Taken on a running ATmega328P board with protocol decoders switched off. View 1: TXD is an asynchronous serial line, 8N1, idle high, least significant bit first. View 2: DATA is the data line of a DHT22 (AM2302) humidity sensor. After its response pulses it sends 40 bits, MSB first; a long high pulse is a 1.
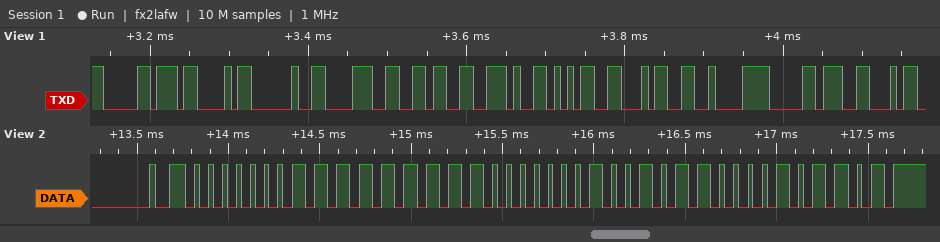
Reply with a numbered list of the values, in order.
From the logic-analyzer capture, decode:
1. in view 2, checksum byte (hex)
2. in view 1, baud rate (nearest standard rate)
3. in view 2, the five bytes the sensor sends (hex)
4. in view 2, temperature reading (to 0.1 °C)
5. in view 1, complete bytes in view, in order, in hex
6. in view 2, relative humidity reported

1. 0x2D
2. 115200 baud
3. 01 FF 01 2C 2D
4. 30.0 °C
5. B0 43 20 38 36 2E 35 34 C2 B0 46
6. 51.1 %
